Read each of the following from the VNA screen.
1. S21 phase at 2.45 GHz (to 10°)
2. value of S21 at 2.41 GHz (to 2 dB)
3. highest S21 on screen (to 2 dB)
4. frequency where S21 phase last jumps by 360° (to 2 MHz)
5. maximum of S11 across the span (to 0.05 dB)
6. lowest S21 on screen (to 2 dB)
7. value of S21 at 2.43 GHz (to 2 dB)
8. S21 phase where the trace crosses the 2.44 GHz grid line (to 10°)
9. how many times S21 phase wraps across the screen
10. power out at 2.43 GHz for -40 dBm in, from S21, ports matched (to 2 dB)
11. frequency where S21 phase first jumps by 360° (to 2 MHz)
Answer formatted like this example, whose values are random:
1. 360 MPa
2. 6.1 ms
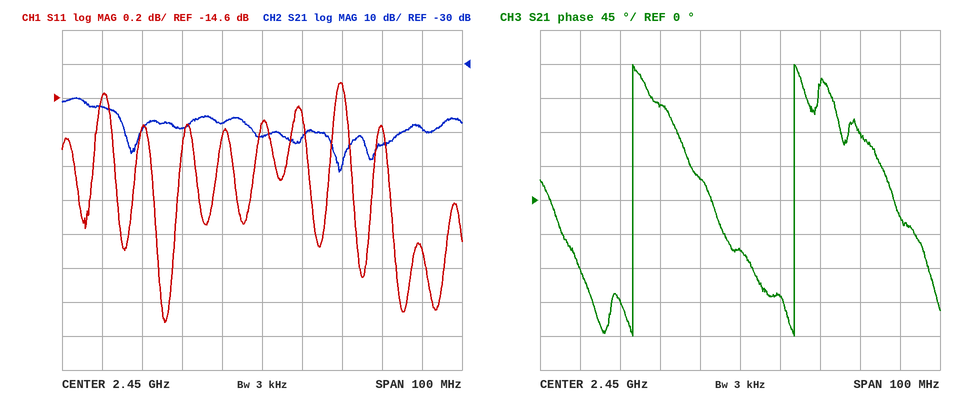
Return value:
1. -70°
2. -42 dB
3. -40 dB
4. 2.464 GHz
5. -14.50 dB
6. -62 dB
7. -48 dB
8. 30°
9. 2
10. -88 dBm
11. 2.424 GHz
